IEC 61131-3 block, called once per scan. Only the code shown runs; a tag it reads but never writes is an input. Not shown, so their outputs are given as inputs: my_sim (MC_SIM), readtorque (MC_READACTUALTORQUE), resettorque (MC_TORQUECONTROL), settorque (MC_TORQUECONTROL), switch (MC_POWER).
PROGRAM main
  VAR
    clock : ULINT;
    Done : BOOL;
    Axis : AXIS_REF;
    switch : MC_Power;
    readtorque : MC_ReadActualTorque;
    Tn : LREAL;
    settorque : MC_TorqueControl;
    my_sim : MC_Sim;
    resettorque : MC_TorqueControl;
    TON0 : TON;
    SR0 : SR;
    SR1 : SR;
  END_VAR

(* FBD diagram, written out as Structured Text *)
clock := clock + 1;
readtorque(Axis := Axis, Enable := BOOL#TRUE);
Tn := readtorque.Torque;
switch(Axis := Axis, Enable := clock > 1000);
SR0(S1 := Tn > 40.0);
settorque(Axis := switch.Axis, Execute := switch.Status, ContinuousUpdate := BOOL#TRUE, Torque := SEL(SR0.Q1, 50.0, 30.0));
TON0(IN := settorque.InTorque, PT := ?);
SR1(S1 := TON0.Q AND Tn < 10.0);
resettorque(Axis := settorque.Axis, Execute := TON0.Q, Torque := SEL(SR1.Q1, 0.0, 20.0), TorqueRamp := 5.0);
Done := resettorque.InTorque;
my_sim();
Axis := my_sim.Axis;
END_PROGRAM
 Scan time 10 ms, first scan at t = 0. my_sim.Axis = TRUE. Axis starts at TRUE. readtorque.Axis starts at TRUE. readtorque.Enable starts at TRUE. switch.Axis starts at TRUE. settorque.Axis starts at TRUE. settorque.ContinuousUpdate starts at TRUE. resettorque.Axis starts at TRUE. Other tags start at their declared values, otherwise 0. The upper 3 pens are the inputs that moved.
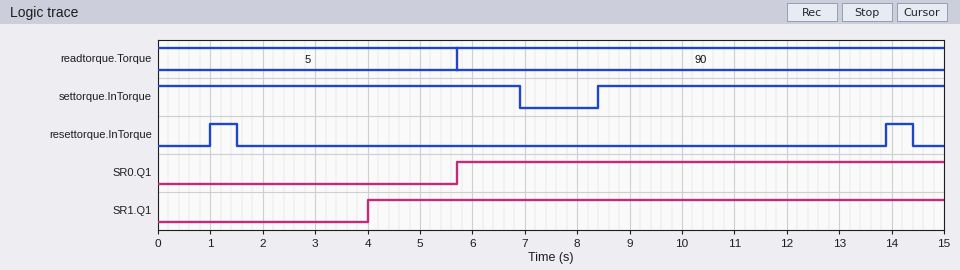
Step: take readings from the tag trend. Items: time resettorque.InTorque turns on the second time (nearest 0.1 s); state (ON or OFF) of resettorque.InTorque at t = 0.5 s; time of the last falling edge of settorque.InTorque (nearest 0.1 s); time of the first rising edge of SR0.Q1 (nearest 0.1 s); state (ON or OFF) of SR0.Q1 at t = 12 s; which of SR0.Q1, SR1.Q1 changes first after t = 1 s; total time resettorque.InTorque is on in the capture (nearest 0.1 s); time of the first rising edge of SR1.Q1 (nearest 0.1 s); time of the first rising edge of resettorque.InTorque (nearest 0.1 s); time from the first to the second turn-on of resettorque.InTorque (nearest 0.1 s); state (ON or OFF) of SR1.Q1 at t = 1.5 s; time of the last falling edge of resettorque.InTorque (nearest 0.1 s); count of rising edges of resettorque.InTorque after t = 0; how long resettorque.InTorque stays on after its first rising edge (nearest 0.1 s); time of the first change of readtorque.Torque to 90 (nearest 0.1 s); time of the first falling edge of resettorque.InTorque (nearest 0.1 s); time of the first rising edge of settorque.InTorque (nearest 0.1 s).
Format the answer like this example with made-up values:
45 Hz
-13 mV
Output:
13.9 s
OFF
6.9 s
5.7 s
ON
SR1.Q1
1.0 s
4.0 s
1.0 s
12.9 s
OFF
14.4 s
2
0.5 s
5.7 s
1.5 s
8.4 s
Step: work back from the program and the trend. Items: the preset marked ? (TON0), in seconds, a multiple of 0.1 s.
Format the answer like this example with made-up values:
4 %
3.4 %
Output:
4.0 s
